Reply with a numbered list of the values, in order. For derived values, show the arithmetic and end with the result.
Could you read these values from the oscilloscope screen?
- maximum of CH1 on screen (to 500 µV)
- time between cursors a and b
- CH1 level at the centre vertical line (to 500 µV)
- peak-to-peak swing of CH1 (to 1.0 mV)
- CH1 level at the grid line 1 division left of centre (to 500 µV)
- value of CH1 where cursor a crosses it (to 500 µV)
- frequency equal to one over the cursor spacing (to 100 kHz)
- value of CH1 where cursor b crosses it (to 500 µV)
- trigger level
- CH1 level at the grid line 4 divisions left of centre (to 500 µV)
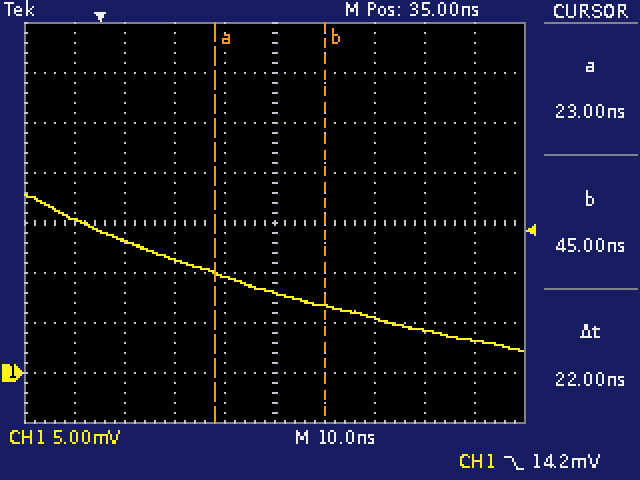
1. 18.0 mV
2. 22 ns
3. 8.0 mV
4. 16.0 mV
5. 9.5 mV
6. 10.0 mV
7. 1 / 22 ns ≈ 45.5 MHz
8. 6.5 mV
9. 14.2 mV
10. 15.5 mV
